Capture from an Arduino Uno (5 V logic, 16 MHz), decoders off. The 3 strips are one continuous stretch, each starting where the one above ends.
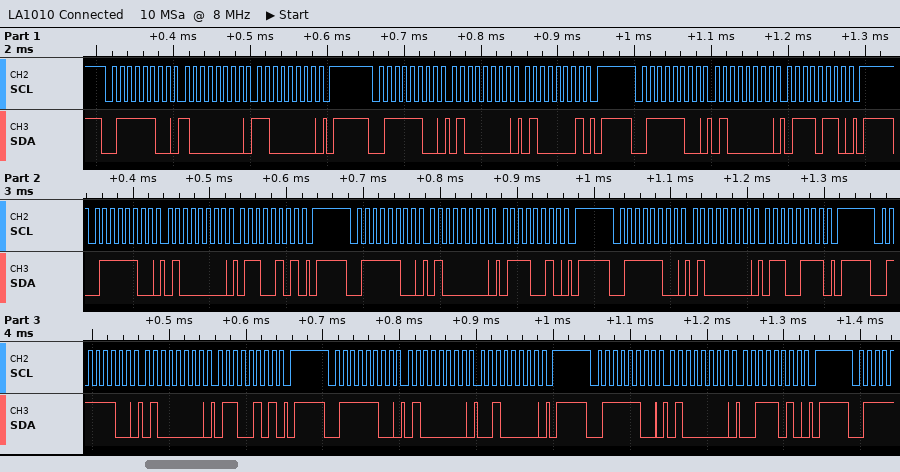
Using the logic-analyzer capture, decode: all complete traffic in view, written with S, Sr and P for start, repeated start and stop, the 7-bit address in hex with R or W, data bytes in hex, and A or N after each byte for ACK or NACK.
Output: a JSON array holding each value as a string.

["S 3EW A 80 A C0 A P S 3EW A 40 A 41 A P S 3EW A 40 A 76 A P S 3EW A 40 A 65 A P S 3EW A 40 A 72 A P S 3EW A 40 A 67 A P S 3EW A 40 A 65 A P S 3EW A 40 A 20 A P S 3EW A 40 A 3A A P"]
